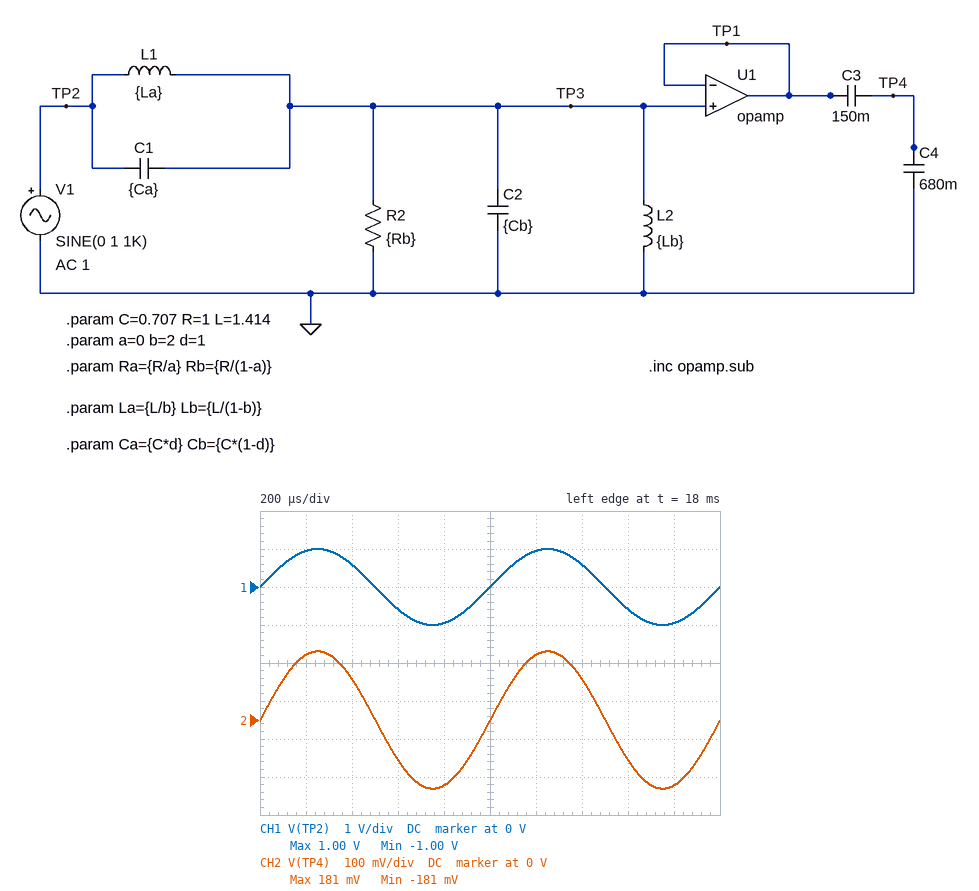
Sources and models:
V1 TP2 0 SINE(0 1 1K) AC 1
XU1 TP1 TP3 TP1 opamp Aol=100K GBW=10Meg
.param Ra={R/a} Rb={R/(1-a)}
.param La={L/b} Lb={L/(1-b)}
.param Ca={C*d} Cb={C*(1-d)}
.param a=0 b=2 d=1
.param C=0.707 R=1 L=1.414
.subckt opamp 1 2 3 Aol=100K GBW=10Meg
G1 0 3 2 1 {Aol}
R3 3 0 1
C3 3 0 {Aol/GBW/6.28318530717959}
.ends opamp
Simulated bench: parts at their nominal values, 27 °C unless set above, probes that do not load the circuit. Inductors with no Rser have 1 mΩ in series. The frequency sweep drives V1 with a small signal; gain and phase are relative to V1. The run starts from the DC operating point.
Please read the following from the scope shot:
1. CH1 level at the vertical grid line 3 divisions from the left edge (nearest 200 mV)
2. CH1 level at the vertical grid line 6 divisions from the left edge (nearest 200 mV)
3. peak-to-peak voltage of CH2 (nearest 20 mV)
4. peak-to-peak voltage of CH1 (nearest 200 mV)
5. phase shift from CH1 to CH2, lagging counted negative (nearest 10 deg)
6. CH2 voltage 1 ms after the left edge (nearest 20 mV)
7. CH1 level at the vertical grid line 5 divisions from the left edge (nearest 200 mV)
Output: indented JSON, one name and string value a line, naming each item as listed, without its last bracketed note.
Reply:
{
  "CH1 level at the vertical grid line 3 divisions from the left edge": "-600 mV",
  "CH1 level at the vertical grid line 6 divisions from the left edge": "1.0 V",
  "peak-to-peak voltage of CH2": "360 mV",
  "peak-to-peak voltage of CH1": "2.0 V",
  "phase shift from CH1 to CH2, lagging counted negative": "0 deg",
  "CH2 voltage 1 ms after the left edge": "0 V",
  "CH1 level at the vertical grid line 5 divisions from the left edge": "0 V"
}
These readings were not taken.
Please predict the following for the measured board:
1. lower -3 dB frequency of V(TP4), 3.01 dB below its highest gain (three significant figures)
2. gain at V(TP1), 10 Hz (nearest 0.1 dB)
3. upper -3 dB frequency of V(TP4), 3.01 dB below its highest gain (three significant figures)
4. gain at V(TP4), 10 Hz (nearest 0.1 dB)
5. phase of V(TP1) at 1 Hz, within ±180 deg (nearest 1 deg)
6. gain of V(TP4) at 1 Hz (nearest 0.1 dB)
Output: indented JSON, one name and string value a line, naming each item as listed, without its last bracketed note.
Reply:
{
  "lower -3 dB frequency of V(TP4), 3.01 dB below its highest gain": "417 µHz",
  "gain at V(TP1), 10 Hz": "0 dB",
  "upper -3 dB frequency of V(TP4), 3.01 dB below its highest gain": "107 mHz",
  "gain at V(TP4), 10 Hz": "-14.9 dB",
  "phase of V(TP1) at 1 Hz, within ±180 deg": "13 deg",
  "gain of V(TP4) at 1 Hz": "-15.3 dB"
}
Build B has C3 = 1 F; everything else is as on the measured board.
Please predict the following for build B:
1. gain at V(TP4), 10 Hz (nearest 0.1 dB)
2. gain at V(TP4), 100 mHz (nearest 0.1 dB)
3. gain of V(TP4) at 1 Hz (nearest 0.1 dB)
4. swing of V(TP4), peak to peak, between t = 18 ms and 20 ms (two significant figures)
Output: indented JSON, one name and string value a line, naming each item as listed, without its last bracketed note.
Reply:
{
  "gain at V(TP4), 10 Hz": "-4.5 dB",
  "gain at V(TP4), 100 mHz": "-1.1 dB",
  "gain of V(TP4) at 1 Hz": "-5.0 dB",
  "swing of V(TP4), peak to peak, between t = 18 ms and 20 ms": "1.2 V"
}
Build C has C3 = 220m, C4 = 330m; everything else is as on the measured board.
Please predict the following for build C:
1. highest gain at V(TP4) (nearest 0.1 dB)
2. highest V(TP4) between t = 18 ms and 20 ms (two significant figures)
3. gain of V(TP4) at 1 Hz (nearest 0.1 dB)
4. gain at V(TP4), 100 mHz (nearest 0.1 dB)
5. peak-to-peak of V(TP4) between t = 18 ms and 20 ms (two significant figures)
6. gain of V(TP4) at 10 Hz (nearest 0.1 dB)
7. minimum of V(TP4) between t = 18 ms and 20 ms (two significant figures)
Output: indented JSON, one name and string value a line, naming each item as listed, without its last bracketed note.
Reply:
{
  "highest gain at V(TP4)": "-2.0 dB",
  "highest V(TP4) between t = 18 ms and 20 ms": "400 mV",
  "gain of V(TP4) at 1 Hz": "-8.4 dB",
  "gain at V(TP4), 100 mHz": "-4.5 dB",
  "peak-to-peak of V(TP4) between t = 18 ms and 20 ms": "800 mV",
  "gain of V(TP4) at 10 Hz": "-8.0 dB",
  "minimum of V(TP4) between t = 18 ms and 20 ms": "-400 mV"
}
